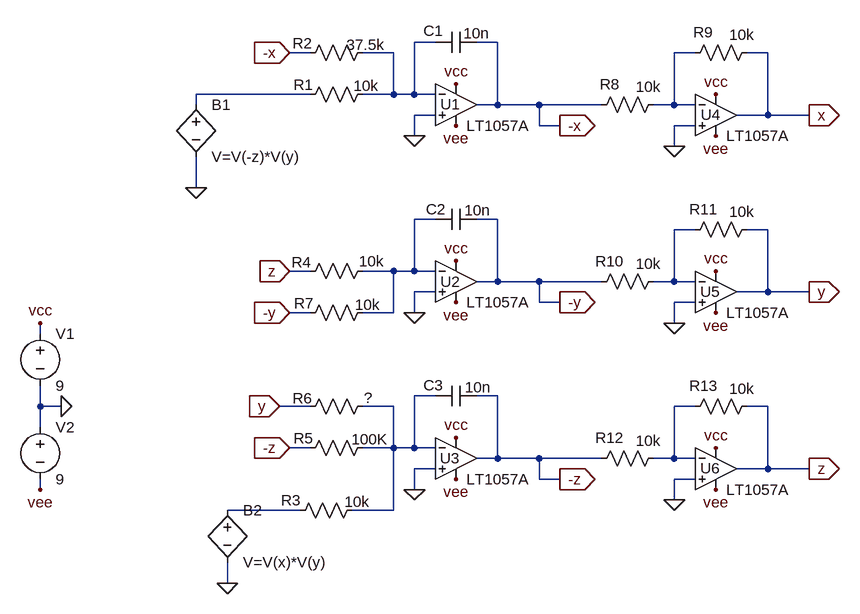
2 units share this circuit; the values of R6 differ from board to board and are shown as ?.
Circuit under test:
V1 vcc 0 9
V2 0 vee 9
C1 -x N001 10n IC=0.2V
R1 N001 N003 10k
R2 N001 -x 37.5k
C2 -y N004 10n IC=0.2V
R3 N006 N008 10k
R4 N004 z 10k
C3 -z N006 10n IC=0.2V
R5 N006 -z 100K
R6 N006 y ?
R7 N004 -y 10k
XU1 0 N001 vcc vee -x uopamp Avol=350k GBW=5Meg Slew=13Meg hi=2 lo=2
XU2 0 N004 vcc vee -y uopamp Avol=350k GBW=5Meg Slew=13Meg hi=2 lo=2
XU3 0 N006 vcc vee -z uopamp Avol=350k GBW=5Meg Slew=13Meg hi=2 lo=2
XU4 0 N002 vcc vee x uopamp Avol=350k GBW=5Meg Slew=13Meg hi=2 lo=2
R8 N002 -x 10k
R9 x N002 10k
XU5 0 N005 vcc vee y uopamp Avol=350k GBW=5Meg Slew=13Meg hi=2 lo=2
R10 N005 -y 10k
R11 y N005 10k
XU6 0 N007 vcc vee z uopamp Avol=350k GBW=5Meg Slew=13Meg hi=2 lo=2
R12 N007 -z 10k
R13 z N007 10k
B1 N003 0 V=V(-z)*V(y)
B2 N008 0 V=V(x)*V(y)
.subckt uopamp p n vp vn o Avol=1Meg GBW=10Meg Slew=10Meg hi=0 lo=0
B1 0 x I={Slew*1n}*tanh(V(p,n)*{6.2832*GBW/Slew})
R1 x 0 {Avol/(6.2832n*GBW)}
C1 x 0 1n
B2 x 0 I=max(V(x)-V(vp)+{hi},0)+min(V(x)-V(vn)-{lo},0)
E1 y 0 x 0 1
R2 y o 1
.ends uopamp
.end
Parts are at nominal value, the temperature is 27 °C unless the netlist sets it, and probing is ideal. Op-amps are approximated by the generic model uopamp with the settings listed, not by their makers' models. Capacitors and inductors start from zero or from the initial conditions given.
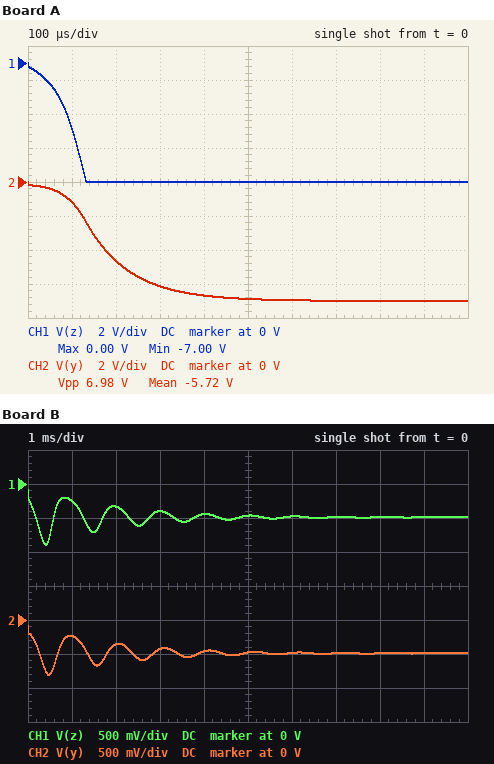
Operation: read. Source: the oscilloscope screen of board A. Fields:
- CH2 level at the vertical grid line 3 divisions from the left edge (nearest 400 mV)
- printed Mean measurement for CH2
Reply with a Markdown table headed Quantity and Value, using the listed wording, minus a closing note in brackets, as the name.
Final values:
| Quantity | Value |
|---|---|
| CH2 level at the vertical grid line 3 divisions from the left edge | -6.0 V |
| printed Mean measurement for CH2 | -5.72 V |
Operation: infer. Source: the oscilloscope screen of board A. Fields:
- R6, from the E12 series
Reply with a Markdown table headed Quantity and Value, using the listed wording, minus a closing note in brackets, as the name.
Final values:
| Quantity | Value |
|---|---|
| R6, from the E12 series | 1.2 kΩ |
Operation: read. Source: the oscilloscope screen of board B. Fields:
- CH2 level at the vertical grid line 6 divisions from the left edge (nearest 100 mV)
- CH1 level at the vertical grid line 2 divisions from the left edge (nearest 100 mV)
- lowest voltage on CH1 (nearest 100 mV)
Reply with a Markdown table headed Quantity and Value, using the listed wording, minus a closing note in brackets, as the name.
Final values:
| Quantity | Value |
|---|---|
| CH2 level at the vertical grid line 6 divisions from the left edge | -500 mV |
| CH1 level at the vertical grid line 2 divisions from the left edge | -300 mV |
| lowest voltage on CH1 | -900 mV |
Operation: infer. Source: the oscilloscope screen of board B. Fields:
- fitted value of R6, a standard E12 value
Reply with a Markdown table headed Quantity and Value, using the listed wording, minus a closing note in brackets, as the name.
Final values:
| Quantity | Value |
|---|---|
| fitted value of R6, a standard E12 value | 10 kΩ |
